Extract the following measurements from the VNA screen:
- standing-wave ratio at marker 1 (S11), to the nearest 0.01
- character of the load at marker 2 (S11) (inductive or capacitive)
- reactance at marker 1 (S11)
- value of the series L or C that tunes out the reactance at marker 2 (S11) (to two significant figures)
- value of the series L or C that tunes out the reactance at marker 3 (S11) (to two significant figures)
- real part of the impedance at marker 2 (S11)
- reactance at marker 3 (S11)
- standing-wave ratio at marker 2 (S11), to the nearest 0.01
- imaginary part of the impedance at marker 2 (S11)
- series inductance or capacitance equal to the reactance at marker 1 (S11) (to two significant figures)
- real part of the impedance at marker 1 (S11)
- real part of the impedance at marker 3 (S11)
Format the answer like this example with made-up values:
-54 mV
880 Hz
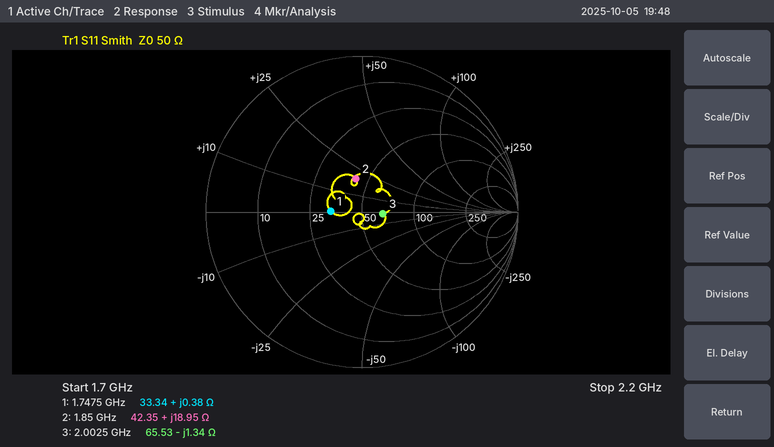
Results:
1.50
inductive
+0.38 Ω
4.5 pF
110 pH
42.35 Ω
-1.34 Ω
1.55
+18.95 Ω
35 pH
33.34 Ω
65.53 Ω
